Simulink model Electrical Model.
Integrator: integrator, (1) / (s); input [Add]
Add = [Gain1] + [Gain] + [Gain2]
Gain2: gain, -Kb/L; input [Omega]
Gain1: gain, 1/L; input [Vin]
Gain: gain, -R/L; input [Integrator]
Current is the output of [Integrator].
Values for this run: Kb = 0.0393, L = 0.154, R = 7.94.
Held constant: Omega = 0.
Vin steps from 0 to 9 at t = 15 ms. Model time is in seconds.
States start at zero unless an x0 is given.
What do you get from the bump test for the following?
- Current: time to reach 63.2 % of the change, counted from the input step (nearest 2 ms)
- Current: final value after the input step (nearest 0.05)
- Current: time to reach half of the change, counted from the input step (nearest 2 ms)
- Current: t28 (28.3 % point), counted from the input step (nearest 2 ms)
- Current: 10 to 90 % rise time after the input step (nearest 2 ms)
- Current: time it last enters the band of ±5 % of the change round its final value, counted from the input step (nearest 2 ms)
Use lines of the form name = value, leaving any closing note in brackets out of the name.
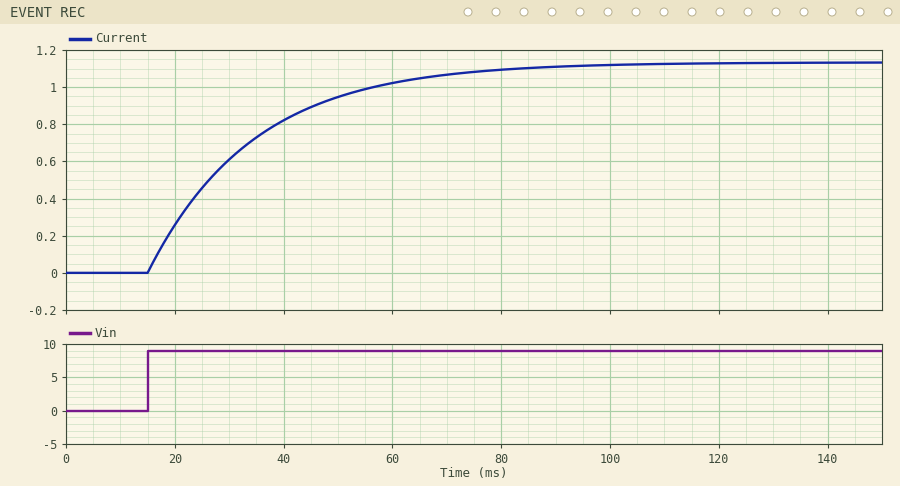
Current: time to reach 63.2 % of the change, counted from the input step = 20 ms
Current: final value after the input step = 1.15
Current: time to reach half of the change, counted from the input step = 14 ms
Current: t28 (28.3 % point), counted from the input step = 6 ms
Current: 10 to 90 % rise time after the input step = 42 ms
Current: time it last enters the band of ±5 % of the change round its final value, counted from the input step = 58 ms
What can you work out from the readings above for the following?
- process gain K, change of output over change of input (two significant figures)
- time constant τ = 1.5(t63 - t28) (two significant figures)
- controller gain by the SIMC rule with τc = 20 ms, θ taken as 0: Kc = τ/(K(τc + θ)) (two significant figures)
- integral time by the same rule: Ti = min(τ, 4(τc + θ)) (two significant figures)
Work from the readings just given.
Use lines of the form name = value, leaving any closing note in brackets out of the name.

process gain K, change of output over change of input = 0.13
time constant τ = 1.5(t63 - t28) = 21 ms
controller gain by the SIMC rule with τc = 20 ms, θ taken as 0: Kc = τ/(K(τc + θ)) = 8.1
integral time by the same rule: Ti = min(τ, 4(τc + θ)) = 21 ms
